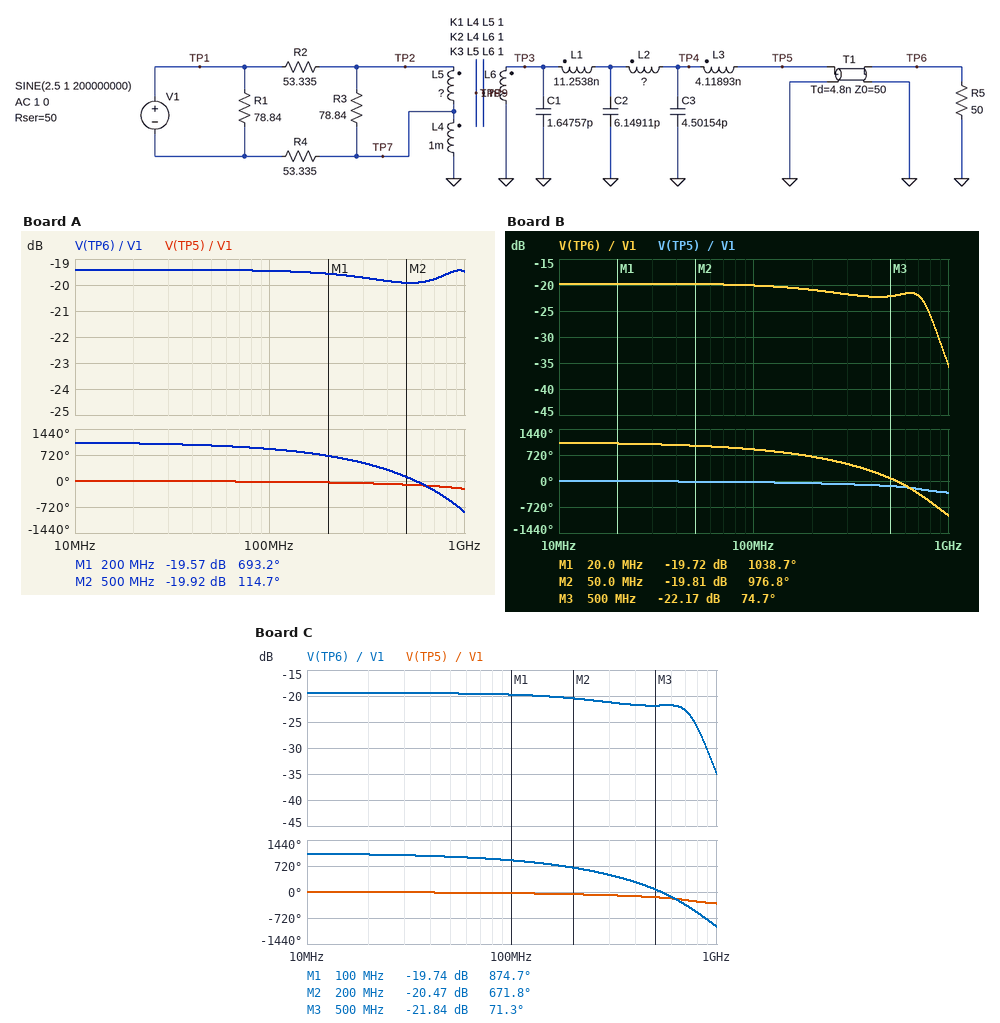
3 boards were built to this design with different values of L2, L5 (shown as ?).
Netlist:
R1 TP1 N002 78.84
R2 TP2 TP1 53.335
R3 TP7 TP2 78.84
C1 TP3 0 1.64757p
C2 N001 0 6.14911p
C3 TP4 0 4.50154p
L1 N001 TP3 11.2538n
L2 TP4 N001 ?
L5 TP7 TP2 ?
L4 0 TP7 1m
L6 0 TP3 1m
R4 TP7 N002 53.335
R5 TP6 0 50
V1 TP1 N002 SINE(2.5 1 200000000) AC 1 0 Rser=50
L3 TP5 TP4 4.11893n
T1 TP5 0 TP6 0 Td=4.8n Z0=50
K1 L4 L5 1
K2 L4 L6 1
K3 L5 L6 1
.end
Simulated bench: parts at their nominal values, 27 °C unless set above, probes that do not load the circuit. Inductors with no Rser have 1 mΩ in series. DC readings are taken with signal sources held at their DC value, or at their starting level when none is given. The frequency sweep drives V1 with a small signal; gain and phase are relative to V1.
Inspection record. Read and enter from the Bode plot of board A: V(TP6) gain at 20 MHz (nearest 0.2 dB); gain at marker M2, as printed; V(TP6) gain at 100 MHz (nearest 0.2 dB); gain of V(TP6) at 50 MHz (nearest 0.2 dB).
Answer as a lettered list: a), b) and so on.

a) -19.4 dB
b) -19.92 dB
c) -19.4 dB
d) -19.4 dB
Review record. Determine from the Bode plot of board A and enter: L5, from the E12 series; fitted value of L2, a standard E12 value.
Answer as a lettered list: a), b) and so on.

a) 560 µH
b) 10 nH
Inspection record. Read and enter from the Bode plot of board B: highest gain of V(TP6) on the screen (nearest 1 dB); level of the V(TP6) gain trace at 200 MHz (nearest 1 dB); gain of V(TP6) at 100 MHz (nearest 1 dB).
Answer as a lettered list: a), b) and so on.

a) -20 dB
b) -21 dB
c) -20 dB
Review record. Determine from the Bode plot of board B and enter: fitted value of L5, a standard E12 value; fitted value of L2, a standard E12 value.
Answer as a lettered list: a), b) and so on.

a) 2.2 mH
b) 39 nH
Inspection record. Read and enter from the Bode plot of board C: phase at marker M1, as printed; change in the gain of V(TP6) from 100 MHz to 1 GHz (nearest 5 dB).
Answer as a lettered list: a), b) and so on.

a) 874.7 deg
b) -15 dB
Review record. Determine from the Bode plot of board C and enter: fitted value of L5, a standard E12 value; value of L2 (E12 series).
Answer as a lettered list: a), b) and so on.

a) 1.8 mH
b) 39 nH
